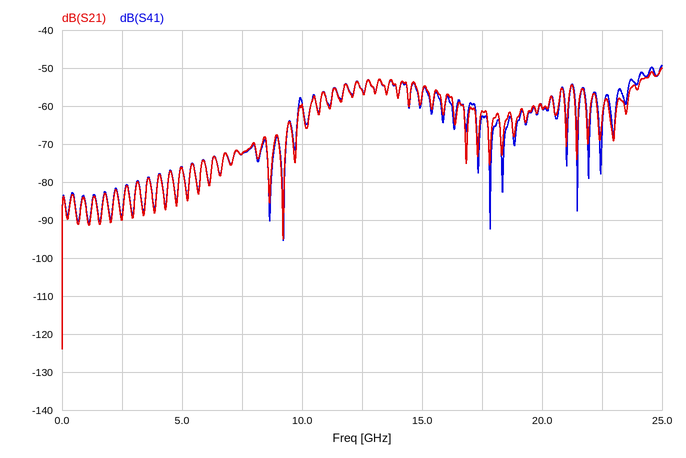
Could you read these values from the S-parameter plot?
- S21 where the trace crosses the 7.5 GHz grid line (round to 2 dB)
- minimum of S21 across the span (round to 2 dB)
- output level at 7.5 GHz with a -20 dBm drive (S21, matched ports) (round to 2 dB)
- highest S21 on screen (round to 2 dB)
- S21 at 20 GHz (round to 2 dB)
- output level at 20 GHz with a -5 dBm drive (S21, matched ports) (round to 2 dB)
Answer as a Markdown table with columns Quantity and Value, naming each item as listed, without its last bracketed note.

| Quantity | Value |
|---|---|
| S21 where the trace crosses the 7.5 GHz grid line | -72 dB |
| minimum of S21 across the span | -124 dB |
| output level at 7.5 GHz with a -20 dBm drive (S21, matched ports) | -92 dBm |
| highest S21 on screen | -50 dB |
| S21 at 20 GHz | -60 dB |
| output level at 20 GHz with a -5 dBm drive (S21, matched ports) | -66 dBm |
